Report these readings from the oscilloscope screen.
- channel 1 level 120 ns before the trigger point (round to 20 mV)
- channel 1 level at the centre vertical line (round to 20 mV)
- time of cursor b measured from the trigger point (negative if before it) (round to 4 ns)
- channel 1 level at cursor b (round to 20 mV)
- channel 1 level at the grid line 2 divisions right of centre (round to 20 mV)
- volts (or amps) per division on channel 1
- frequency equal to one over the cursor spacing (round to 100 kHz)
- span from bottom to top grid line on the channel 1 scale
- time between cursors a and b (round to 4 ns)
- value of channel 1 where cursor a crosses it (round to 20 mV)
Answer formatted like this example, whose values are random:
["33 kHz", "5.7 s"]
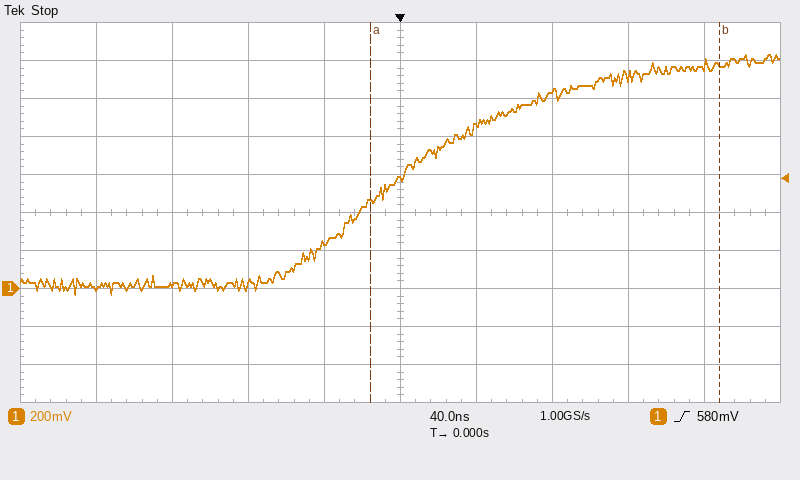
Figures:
["20 mV", "580 mV", "+168 ns", "1.18 V", "1.04 V", "200 mV", "5.4 MHz", "2 V", "184 ns", "460 mV"]
